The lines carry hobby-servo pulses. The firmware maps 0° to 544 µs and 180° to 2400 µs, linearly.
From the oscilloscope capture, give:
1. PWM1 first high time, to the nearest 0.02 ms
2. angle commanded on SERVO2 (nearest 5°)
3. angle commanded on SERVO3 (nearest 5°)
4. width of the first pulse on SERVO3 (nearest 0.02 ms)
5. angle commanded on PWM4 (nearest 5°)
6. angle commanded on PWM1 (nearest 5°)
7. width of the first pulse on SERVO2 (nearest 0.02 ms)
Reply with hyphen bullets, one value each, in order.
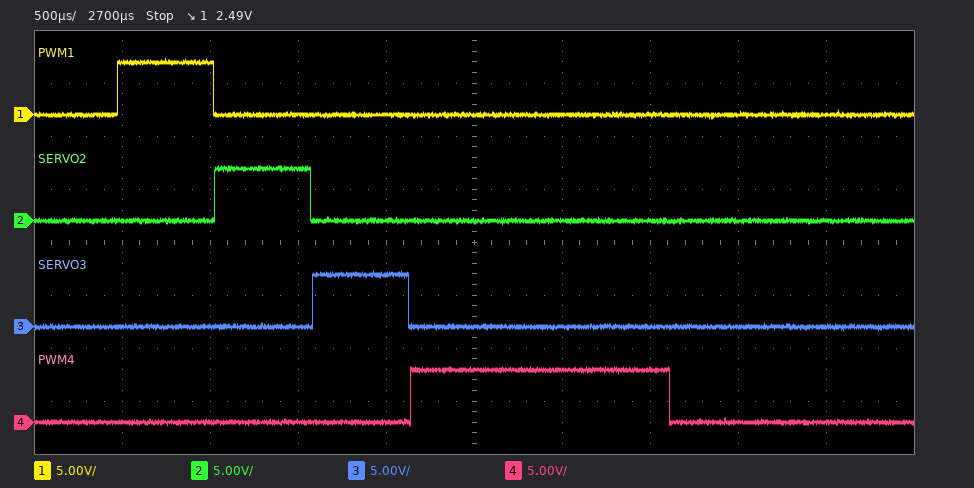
- 0.54 ms
- 0°
- 0°
- 0.54 ms
- 90°
- 0°
- 0.54 ms
